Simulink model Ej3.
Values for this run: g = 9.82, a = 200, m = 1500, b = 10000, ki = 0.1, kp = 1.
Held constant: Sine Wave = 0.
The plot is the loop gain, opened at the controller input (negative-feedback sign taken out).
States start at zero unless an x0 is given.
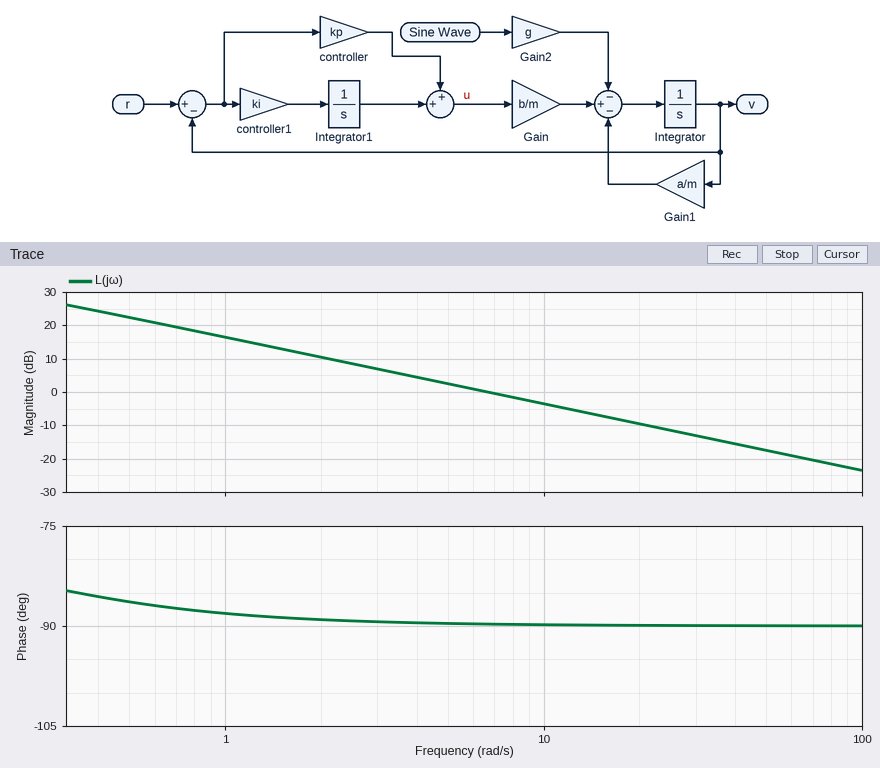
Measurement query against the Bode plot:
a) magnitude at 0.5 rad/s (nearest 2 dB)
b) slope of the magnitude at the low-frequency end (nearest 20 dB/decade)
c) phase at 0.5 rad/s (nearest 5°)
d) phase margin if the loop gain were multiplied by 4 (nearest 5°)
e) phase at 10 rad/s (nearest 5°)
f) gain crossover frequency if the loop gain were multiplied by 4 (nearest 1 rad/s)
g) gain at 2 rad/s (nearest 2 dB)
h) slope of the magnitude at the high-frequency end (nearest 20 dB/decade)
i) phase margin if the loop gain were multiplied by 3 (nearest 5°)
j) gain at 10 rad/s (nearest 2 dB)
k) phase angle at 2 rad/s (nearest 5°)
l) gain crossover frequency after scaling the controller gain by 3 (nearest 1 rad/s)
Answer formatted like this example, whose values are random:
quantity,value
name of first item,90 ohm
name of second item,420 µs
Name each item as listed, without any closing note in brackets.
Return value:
quantity,value
magnitude at 0.5 rad/s,22 dB
slope of the magnitude at the low-frequency end,-20 dB/decade
phase at 0.5 rad/s,-85°
phase margin if the loop gain were multiplied by 4,90°
phase at 10 rad/s,-90°
gain crossover frequency if the loop gain were multiplied by 4,27 rad/s
gain at 2 rad/s,10 dB
slope of the magnitude at the high-frequency end,-20 dB/decade
phase margin if the loop gain were multiplied by 3,90°
gain at 10 rad/s,-4 dB
phase angle at 2 rad/s,-90°
gain crossover frequency after scaling the controller gain by 3,20 rad/s
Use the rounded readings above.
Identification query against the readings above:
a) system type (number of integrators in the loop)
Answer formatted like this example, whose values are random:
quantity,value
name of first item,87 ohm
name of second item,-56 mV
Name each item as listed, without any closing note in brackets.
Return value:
quantity,value
system type,1
